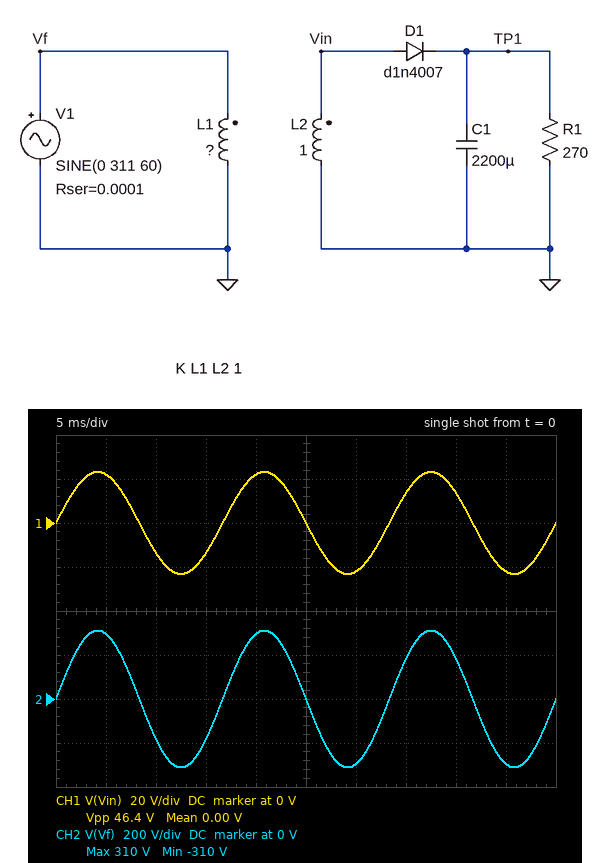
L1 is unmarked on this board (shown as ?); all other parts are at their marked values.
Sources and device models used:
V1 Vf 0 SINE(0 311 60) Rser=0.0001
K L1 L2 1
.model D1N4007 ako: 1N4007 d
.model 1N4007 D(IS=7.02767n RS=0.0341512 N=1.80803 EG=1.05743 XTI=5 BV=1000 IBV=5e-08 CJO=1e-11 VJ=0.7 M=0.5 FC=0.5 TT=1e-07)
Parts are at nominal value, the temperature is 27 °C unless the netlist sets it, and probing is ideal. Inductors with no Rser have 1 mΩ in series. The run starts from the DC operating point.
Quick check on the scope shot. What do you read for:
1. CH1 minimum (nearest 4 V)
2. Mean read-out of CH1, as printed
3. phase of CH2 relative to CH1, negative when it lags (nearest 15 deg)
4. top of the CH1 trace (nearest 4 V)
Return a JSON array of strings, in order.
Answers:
["-24 V", "0.00 V", "0 deg", "24 V"]
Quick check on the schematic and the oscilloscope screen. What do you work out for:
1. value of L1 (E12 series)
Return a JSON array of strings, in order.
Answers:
["180 H"]
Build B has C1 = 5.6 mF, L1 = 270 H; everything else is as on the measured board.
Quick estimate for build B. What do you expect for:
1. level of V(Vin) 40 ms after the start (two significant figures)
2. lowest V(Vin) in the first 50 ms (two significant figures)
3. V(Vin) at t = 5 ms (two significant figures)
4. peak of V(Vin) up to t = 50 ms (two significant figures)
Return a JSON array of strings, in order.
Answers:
["11 V", "-19 V", "18 V", "19 V"]
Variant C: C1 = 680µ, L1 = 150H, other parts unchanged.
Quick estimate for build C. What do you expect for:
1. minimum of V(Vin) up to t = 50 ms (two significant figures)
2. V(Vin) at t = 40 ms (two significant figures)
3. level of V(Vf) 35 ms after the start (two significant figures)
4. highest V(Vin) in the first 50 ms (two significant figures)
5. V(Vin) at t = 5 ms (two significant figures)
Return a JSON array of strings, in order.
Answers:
["-25 V", "15 V", "180 V", "25 V", "24 V"]
